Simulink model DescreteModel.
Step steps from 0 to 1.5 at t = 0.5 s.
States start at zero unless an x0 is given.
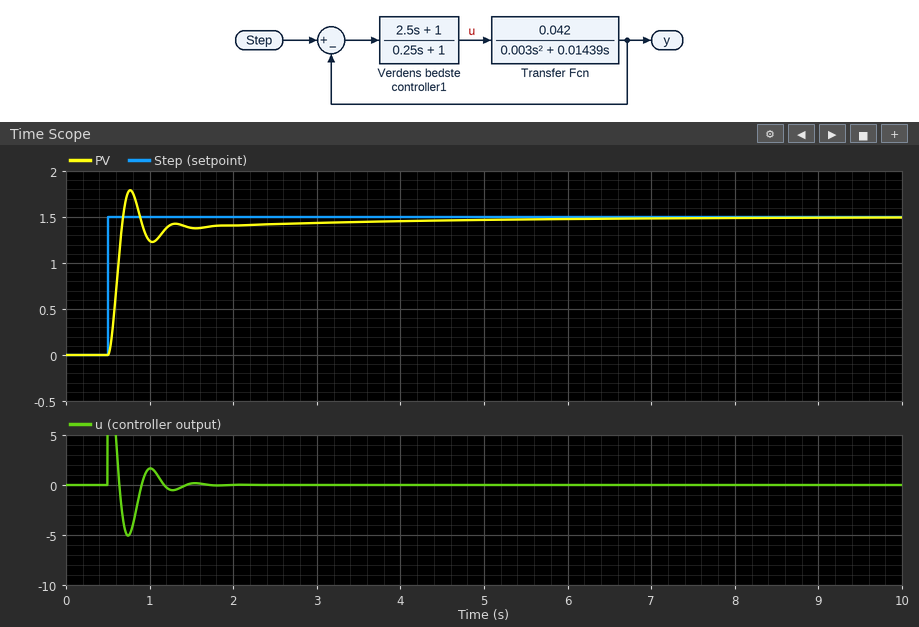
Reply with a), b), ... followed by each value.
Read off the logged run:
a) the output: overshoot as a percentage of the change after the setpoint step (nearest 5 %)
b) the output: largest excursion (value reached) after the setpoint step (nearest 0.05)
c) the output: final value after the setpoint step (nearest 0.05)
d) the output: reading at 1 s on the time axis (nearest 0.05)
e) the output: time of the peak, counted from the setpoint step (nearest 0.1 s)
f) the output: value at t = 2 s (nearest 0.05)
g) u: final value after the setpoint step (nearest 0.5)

a) 20 %
b) 1.80
c) 1.50
d) 1.25
e) 0.3 s
f) 1.40
g) 0.0
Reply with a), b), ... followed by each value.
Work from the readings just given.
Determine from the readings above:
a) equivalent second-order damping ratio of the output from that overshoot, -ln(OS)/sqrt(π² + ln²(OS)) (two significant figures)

a) 0.46
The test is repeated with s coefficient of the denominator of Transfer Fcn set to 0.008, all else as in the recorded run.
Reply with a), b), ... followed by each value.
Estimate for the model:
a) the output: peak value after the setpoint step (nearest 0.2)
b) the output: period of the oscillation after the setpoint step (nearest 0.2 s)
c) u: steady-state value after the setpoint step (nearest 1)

a) 2.0
b) 0.6 s
c) 0
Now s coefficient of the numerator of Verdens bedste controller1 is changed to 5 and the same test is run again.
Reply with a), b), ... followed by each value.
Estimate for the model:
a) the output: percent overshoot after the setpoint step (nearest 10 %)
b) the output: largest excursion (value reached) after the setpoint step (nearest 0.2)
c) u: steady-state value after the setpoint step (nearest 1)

a) 40 %
b) 2.0
c) 0
